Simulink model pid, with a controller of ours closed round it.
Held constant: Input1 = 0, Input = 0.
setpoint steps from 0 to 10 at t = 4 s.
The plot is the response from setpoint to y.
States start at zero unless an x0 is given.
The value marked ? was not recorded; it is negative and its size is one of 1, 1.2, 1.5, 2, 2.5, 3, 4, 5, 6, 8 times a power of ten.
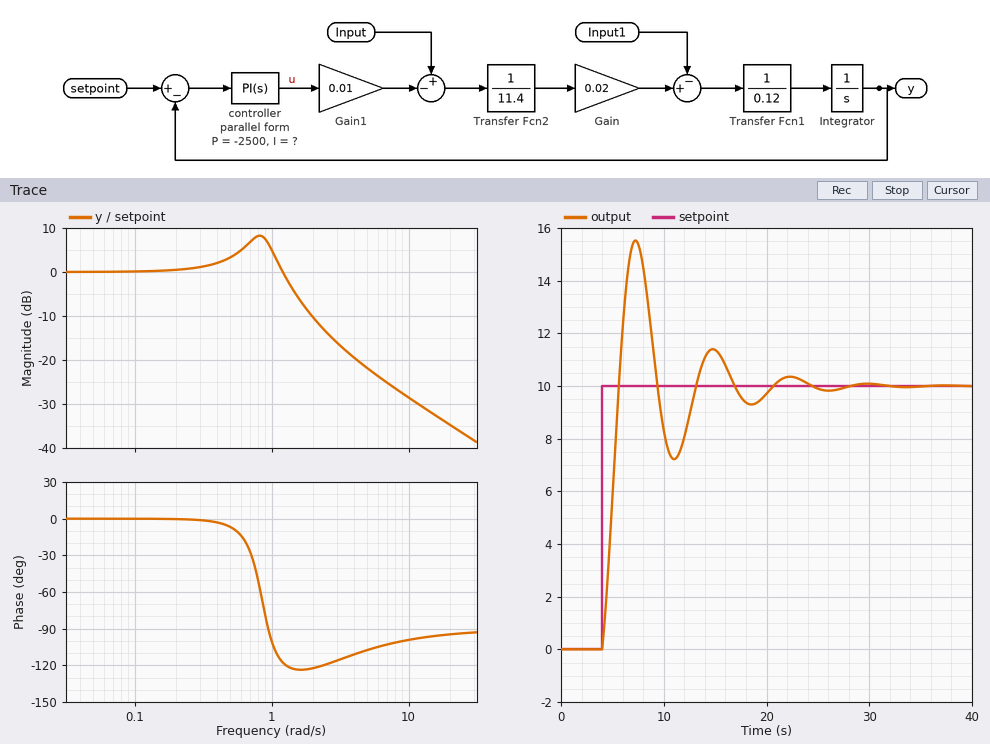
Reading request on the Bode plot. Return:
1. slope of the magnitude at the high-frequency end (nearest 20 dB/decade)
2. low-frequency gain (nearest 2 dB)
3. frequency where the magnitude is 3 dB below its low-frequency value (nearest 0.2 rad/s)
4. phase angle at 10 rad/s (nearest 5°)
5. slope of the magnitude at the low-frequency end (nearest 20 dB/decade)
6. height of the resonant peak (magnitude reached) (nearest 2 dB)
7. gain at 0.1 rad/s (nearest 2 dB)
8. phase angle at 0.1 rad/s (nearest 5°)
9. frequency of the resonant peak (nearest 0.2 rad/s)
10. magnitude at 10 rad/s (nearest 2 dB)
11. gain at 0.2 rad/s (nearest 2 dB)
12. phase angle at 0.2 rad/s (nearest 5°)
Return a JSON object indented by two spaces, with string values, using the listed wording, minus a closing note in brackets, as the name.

{
  "slope of the magnitude at the high-frequency end": "-20 dB/decade",
  "low-frequency gain": "0 dB",
  "frequency where the magnitude is 3 dB below its low-frequency value": "1.4 rad/s",
  "phase angle at 10 rad/s": "-100°",
  "slope of the magnitude at the low-frequency end": "0 dB/decade",
  "height of the resonant peak (magnitude reached)": "8 dB",
  "gain at 0.1 rad/s": "0 dB",
  "phase angle at 0.1 rad/s": "0°",
  "frequency of the resonant peak": "0.8 rad/s",
  "magnitude at 10 rad/s": "-28 dB",
  "gain at 0.2 rad/s": "0 dB",
  "phase angle at 0.2 rad/s": "0°"
}
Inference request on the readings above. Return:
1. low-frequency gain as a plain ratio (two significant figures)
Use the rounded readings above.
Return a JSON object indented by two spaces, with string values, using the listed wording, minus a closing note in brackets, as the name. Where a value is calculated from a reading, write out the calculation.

{
  "low-frequency gain as a plain ratio": "10^(0 / 20) = 1.0"
}
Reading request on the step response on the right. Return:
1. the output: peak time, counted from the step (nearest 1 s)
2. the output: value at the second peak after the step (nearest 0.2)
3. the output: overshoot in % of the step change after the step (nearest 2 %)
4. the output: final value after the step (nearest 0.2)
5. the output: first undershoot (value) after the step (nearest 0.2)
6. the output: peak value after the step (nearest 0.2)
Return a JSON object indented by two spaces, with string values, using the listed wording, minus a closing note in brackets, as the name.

{
  "the output: peak time, counted from the step": "3 s",
  "the output: value at the second peak after the step": "11.4",
  "the output: overshoot in % of the step change after the step": "56 %",
  "the output: final value after the step": "10.0",
  "the output: first undershoot (value) after the step": "7.2",
  "the output: peak value after the step": "15.6"
}
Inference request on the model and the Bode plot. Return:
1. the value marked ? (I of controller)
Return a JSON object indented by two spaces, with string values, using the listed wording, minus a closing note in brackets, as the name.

{
  "the value marked ?": "-5000"
}
